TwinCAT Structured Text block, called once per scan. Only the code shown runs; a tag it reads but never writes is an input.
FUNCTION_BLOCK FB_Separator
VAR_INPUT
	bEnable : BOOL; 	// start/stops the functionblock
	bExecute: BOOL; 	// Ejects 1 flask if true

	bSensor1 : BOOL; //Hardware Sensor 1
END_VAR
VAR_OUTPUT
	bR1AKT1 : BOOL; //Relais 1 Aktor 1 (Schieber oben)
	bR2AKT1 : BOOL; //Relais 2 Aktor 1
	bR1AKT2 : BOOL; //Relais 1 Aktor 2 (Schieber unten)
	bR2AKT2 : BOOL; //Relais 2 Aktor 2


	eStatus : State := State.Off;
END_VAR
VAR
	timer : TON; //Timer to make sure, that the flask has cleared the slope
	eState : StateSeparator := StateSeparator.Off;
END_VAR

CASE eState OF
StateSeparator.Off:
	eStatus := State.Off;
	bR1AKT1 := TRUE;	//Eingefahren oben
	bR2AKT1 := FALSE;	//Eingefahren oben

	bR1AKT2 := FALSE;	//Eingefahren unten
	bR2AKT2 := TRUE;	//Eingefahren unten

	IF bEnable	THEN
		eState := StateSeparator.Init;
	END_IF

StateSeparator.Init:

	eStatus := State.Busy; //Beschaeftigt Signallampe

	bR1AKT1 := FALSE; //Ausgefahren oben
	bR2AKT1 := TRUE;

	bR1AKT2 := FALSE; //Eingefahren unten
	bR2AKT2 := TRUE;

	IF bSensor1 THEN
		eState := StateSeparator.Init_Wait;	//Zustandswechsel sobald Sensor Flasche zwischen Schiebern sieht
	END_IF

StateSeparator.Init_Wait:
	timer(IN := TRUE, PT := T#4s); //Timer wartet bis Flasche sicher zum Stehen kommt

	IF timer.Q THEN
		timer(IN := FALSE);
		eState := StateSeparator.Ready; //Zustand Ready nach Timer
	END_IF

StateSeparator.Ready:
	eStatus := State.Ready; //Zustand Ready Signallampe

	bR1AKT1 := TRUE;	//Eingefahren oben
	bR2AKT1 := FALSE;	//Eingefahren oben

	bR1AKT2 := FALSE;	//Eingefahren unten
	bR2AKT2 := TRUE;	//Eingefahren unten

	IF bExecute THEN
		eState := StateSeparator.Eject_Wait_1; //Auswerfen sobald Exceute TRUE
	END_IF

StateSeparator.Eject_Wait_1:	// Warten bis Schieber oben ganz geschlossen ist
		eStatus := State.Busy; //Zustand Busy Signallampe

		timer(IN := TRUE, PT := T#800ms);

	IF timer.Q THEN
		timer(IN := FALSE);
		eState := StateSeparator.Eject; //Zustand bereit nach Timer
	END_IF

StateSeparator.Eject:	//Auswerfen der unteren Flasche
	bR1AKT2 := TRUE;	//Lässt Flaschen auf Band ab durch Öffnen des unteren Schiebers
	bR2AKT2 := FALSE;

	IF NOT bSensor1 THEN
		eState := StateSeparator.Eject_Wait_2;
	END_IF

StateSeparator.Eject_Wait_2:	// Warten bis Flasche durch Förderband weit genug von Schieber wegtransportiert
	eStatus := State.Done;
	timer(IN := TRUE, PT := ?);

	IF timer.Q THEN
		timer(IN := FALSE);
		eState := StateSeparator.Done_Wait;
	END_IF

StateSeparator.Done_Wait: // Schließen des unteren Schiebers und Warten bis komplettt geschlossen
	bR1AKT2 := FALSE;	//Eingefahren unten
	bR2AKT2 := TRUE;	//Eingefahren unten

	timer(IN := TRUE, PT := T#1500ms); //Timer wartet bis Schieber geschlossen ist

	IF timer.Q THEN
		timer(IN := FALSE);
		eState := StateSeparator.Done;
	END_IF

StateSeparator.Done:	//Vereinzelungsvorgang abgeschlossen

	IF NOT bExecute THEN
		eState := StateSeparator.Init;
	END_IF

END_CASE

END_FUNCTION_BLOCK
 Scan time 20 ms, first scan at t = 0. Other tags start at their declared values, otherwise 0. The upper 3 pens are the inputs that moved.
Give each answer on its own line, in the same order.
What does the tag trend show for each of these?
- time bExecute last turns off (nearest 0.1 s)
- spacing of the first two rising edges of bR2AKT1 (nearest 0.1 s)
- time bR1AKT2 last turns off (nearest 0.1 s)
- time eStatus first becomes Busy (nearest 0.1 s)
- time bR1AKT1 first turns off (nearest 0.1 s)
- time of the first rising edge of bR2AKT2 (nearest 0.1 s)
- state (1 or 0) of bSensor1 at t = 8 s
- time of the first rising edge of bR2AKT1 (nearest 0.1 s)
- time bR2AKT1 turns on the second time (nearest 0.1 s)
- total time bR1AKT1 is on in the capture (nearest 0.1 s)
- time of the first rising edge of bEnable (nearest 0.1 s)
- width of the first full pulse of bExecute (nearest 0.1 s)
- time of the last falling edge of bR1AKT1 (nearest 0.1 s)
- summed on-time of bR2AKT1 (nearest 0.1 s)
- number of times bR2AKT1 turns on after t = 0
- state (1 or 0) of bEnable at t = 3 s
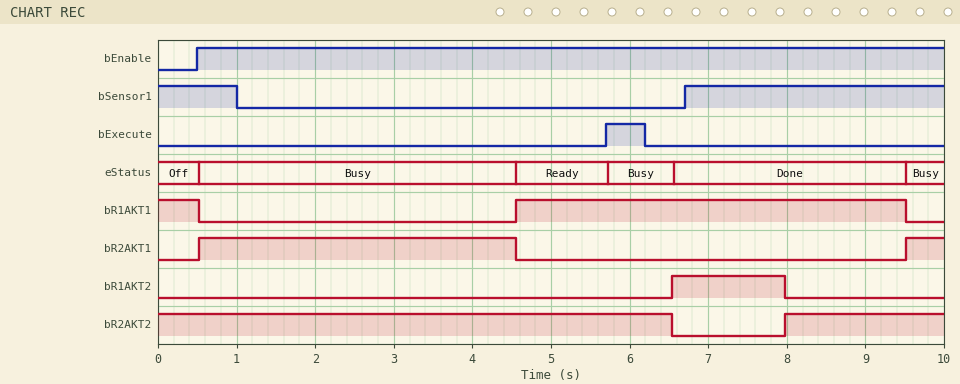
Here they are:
6.2 s
9.0 s
8.0 s
0.5 s
0.5 s
8.0 s
1
0.5 s
9.5 s
5.5 s
0.5 s
0.5 s
9.5 s
4.5 s
2
1
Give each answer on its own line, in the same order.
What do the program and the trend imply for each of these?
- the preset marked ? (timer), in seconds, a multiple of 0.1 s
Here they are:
1.4 s
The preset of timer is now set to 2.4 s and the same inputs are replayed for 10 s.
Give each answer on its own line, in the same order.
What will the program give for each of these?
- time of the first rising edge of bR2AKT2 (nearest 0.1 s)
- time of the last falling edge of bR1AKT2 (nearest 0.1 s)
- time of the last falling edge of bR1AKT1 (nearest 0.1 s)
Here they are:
9.0 s
9.0 s
0.5 s
